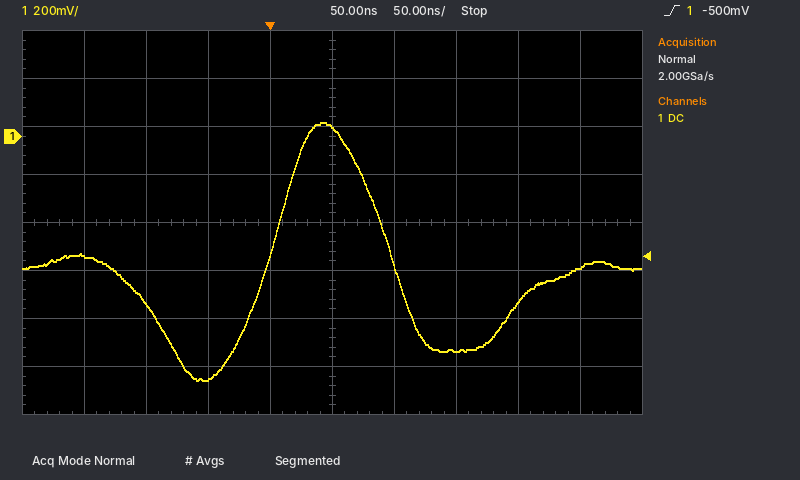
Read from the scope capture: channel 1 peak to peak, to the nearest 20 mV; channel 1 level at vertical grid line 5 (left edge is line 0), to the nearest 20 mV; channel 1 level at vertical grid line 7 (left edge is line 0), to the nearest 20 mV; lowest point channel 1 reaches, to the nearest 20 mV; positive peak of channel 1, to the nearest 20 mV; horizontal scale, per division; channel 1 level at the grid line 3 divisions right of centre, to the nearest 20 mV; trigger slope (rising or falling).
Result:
1.08 V
40 mV
-900 mV
-1.02 V
60 mV
50 ns
-700 mV
rising
